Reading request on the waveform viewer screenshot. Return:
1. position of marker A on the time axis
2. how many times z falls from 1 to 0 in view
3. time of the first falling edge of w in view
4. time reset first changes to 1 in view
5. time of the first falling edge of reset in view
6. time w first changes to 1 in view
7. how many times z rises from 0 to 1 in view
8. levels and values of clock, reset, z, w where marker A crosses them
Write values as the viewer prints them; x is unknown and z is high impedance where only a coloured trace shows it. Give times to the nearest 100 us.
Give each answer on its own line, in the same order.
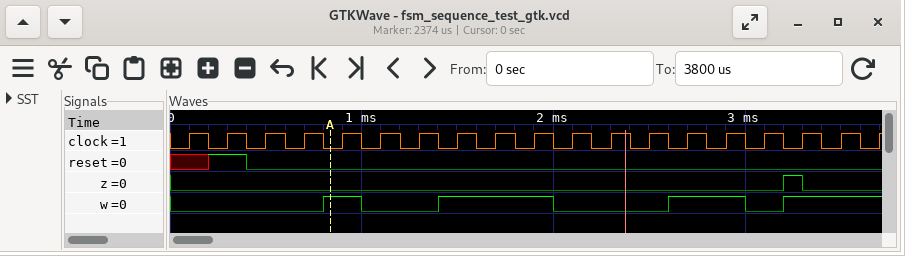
800 us
1
1000 us
200 us
400 us
800 us
1
clock=0, reset=0, z=0, w=1
